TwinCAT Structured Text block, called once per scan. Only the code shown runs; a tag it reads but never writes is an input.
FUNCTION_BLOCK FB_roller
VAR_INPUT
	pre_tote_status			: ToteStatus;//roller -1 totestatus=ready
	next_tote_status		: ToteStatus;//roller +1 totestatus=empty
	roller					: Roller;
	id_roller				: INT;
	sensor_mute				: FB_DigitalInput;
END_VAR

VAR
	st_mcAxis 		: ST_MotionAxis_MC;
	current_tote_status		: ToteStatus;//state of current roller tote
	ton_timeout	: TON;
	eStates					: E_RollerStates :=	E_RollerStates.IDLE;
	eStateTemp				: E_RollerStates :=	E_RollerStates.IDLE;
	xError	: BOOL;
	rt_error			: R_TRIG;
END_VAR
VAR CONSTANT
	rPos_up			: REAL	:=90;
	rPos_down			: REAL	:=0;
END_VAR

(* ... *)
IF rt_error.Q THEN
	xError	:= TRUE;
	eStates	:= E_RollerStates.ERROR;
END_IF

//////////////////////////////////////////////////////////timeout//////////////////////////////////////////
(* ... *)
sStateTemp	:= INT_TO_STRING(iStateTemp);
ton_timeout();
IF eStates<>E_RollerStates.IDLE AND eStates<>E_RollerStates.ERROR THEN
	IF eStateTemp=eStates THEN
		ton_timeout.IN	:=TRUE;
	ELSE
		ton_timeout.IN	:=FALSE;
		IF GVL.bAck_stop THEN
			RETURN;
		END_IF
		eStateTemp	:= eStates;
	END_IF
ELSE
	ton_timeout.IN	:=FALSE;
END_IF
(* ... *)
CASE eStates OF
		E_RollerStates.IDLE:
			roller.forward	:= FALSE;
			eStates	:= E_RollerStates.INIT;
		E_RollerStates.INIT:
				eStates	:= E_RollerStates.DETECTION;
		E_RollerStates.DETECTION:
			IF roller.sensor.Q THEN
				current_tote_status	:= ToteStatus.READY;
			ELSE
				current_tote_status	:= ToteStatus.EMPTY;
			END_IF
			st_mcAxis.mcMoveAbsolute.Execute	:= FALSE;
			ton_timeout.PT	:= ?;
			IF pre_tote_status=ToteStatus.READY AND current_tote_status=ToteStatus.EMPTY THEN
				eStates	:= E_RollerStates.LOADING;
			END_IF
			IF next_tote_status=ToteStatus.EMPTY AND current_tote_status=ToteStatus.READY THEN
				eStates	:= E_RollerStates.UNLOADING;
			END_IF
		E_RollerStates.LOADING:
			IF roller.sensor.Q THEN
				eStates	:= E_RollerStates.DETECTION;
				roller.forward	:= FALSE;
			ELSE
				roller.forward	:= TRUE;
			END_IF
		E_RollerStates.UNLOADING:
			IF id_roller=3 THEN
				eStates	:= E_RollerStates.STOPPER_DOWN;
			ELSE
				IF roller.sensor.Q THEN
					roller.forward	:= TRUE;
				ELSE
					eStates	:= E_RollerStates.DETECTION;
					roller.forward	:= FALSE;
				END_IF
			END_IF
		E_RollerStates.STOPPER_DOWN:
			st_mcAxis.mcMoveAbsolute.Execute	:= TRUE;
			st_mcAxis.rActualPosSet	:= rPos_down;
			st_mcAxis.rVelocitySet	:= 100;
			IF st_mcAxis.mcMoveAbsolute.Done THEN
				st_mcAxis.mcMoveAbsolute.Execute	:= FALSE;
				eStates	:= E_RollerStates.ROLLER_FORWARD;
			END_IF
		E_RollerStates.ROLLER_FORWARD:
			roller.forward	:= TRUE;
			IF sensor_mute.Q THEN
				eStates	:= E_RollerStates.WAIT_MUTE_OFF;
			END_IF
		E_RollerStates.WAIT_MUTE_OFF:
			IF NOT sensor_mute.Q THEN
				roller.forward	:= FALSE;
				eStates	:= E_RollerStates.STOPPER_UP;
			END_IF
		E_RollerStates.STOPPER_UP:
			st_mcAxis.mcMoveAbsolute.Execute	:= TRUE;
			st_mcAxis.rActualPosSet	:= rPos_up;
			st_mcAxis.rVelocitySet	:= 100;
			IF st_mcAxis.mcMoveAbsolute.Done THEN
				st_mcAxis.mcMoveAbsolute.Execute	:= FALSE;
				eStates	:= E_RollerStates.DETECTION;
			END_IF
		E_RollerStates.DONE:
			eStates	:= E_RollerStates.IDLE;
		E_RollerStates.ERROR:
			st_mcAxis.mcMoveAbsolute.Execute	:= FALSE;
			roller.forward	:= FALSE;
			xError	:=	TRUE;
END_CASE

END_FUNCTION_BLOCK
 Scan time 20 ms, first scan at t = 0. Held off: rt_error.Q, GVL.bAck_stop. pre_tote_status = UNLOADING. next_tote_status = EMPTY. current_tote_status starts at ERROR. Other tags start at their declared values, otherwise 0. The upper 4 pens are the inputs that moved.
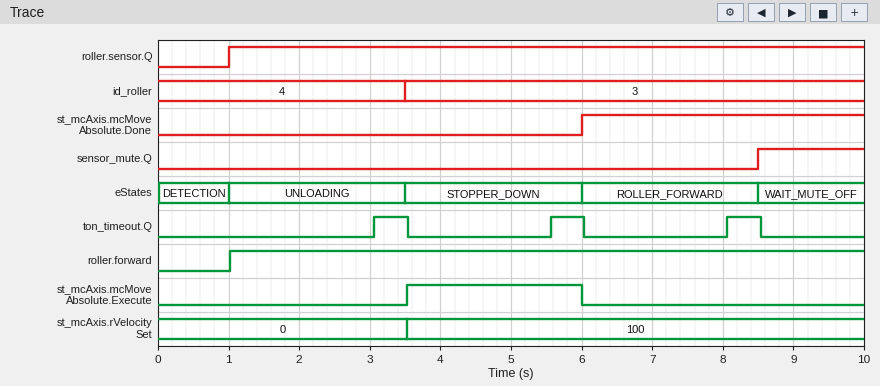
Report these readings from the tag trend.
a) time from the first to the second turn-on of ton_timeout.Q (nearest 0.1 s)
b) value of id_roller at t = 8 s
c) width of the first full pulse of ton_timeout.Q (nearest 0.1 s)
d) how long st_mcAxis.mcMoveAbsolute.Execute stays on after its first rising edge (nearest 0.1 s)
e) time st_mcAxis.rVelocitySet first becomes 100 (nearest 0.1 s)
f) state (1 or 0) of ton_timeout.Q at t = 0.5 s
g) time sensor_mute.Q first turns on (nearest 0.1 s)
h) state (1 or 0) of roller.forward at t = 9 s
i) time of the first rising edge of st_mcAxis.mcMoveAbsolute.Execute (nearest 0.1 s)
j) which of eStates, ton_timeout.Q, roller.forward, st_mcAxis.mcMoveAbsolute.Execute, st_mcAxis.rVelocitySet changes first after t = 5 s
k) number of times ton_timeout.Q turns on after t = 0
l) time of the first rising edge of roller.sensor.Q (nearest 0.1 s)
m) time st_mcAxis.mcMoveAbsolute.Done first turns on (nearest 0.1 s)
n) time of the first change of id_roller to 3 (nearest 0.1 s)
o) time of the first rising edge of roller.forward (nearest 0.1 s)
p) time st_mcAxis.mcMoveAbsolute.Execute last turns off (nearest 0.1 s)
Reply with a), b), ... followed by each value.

a) 2.5 s
b) 3
c) 0.5 s
d) 2.5 s
e) 3.5 s
f) 0
g) 8.5 s
h) 1
i) 3.5 s
j) ton_timeout.Q
k) 3
l) 1.0 s
m) 6.0 s
n) 3.5 s
o) 1.0 s
p) 6.0 s
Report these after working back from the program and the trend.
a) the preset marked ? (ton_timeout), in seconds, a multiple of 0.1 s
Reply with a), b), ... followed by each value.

a) 2.0 s
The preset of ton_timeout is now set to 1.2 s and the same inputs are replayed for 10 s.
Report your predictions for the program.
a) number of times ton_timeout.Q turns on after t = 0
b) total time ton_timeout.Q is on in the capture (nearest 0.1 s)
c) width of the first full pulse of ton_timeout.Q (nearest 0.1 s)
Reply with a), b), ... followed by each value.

a) 4
b) 4.1 s
c) 1.3 s
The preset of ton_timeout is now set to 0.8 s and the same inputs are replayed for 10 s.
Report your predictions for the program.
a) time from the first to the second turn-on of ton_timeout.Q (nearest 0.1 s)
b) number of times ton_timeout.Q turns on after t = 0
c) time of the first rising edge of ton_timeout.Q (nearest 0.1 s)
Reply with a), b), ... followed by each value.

a) 1.0 s
b) 5
c) 0.9 s
